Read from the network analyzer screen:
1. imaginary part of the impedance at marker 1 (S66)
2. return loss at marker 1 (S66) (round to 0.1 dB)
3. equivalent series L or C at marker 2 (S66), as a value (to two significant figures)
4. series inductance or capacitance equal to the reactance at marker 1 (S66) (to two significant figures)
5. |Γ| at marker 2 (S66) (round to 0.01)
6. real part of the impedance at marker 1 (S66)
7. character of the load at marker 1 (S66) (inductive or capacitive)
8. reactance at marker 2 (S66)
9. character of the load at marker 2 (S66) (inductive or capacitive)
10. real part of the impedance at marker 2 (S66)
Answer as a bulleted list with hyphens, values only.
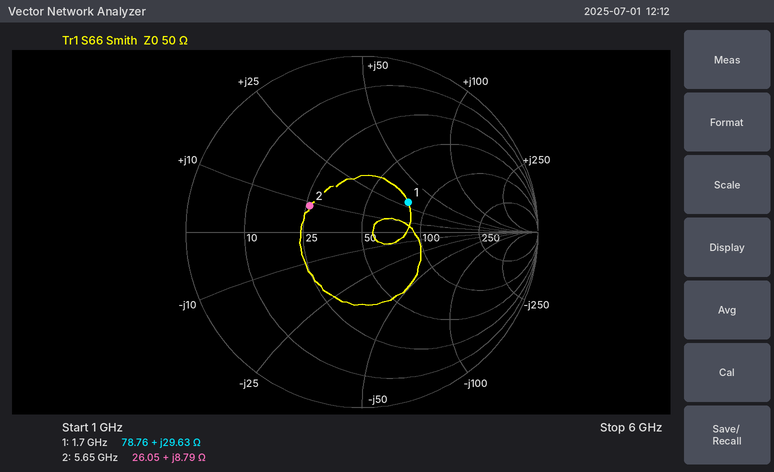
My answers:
- +29.63 Ω
- 10.1 dB
- 250 pH
- 2.8 nH
- 0.33
- 78.76 Ω
- inductive
- +8.79 Ω
- inductive
- 26.05 Ω
